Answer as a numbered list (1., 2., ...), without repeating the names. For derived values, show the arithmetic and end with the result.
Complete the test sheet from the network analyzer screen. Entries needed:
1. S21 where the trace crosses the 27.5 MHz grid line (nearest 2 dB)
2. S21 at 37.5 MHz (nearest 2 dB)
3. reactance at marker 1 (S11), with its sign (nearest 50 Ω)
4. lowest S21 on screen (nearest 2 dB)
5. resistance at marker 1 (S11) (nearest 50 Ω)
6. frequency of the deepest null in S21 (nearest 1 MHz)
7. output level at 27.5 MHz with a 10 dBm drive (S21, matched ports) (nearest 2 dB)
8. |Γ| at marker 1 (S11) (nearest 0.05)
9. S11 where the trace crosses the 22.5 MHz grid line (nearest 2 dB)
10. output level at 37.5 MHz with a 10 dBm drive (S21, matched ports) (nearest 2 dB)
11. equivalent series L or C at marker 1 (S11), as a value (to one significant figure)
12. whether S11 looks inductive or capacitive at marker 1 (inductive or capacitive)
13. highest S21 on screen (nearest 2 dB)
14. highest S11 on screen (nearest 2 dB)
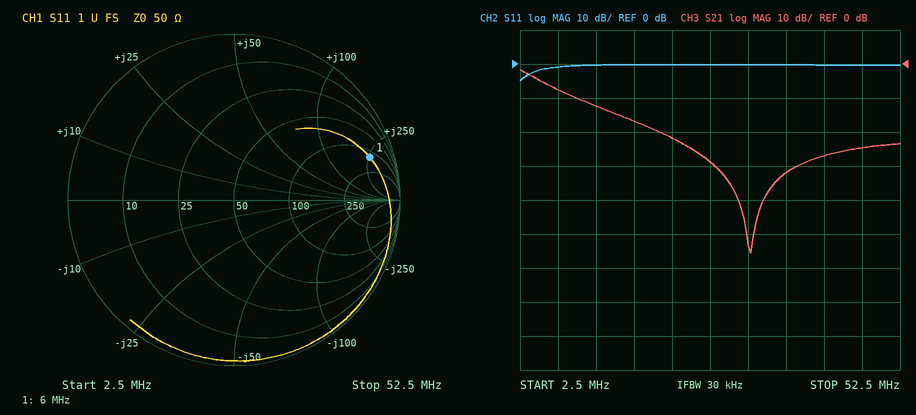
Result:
1. -28 dB
2. -32 dB
3. +250 Ω
4. -56 dB
5. 150 Ω
6. 33 MHz
7. 10 dBm + (-28 dB) = -18 dBm
8. 0.85
9. 0 dB
10. 10 dBm + (-32 dB) = -22 dBm
11. L = 250 Ω/(2π × 6 MHz) ≈ 7 µH
12. inductive
13. -2 dB
14. 0 dB
